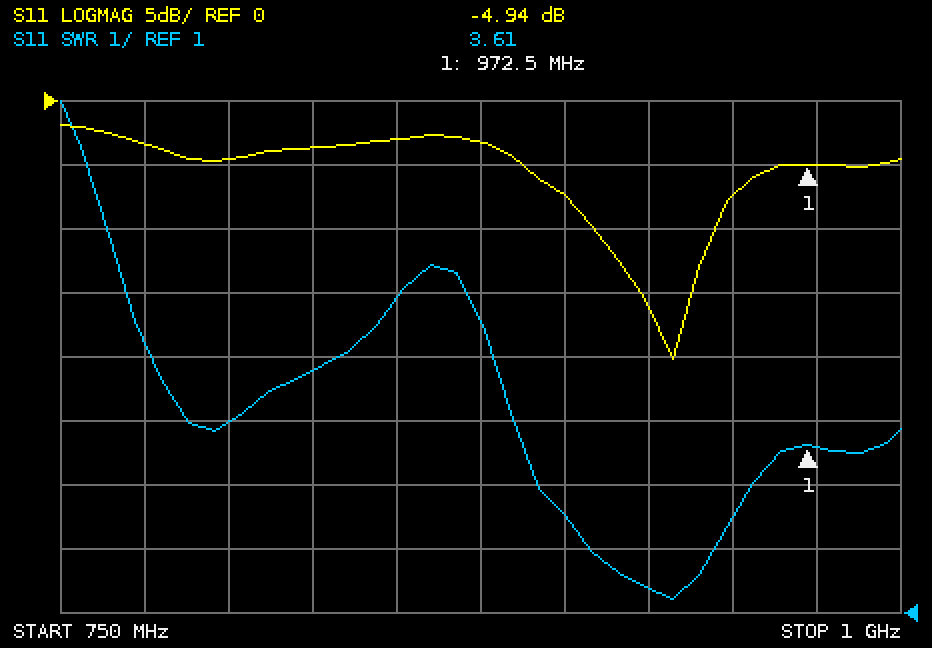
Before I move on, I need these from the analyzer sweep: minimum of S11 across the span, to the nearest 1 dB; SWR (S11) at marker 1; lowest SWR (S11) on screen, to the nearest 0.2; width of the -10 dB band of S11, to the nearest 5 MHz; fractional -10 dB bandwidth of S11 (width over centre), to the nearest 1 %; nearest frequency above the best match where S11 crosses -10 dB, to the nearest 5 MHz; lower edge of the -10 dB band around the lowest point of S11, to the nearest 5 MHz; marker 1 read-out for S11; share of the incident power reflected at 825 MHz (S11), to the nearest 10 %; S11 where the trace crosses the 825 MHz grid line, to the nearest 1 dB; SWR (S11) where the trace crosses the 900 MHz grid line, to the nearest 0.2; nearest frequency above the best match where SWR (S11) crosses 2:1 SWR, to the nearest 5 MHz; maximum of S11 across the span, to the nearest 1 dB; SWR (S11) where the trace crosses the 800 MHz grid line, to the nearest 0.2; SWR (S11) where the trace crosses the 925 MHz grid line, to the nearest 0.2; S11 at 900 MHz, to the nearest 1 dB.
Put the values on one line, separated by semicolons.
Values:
-20 dB; 3.61; 1.2; 35 MHz; 4 %; 945 MHz; 910 MHz; -4.94 dB; 40 %; -4 dB; 2.6; 945 MHz; -2 dB; 4.0; 1.4; -7 dB
